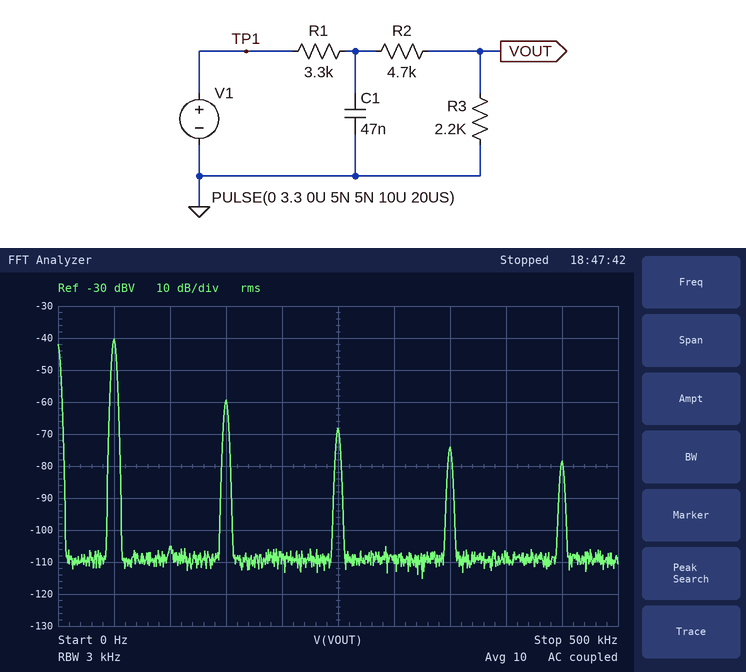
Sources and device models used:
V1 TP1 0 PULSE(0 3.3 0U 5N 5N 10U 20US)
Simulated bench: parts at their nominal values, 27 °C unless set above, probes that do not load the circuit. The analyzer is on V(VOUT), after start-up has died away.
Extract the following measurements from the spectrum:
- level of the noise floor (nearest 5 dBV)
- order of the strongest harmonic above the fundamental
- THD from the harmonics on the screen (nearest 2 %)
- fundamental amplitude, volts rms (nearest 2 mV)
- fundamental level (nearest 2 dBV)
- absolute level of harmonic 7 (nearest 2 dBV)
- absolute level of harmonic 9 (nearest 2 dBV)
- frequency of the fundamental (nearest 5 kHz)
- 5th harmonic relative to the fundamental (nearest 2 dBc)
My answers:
-110 dBV
3
12 %
10 mV
-40 dBV
-74 dBV
-78 dBV
50 kHz
-28 dBc
